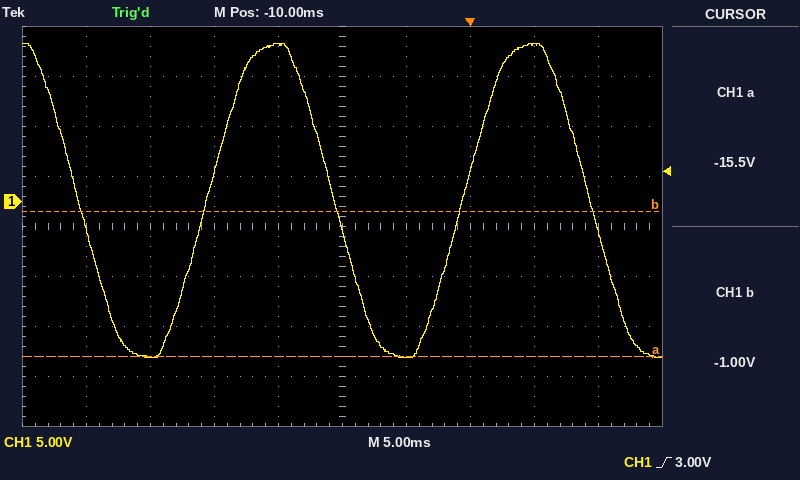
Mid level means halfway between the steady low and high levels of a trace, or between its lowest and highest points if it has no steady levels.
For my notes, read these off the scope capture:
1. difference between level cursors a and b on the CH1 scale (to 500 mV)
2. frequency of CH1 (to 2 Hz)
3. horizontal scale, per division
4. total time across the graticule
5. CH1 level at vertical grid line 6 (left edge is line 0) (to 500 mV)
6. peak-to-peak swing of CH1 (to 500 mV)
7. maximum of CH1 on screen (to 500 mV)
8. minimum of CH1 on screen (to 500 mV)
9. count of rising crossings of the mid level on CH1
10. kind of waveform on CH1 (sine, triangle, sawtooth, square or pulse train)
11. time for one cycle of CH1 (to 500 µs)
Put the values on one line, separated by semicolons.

14.5 V; 50 Hz; 5 ms; 50 ms; -15.5 V; 31.5 V; 16.0 V; -15.5 V; 2; sine; 20.0 ms
